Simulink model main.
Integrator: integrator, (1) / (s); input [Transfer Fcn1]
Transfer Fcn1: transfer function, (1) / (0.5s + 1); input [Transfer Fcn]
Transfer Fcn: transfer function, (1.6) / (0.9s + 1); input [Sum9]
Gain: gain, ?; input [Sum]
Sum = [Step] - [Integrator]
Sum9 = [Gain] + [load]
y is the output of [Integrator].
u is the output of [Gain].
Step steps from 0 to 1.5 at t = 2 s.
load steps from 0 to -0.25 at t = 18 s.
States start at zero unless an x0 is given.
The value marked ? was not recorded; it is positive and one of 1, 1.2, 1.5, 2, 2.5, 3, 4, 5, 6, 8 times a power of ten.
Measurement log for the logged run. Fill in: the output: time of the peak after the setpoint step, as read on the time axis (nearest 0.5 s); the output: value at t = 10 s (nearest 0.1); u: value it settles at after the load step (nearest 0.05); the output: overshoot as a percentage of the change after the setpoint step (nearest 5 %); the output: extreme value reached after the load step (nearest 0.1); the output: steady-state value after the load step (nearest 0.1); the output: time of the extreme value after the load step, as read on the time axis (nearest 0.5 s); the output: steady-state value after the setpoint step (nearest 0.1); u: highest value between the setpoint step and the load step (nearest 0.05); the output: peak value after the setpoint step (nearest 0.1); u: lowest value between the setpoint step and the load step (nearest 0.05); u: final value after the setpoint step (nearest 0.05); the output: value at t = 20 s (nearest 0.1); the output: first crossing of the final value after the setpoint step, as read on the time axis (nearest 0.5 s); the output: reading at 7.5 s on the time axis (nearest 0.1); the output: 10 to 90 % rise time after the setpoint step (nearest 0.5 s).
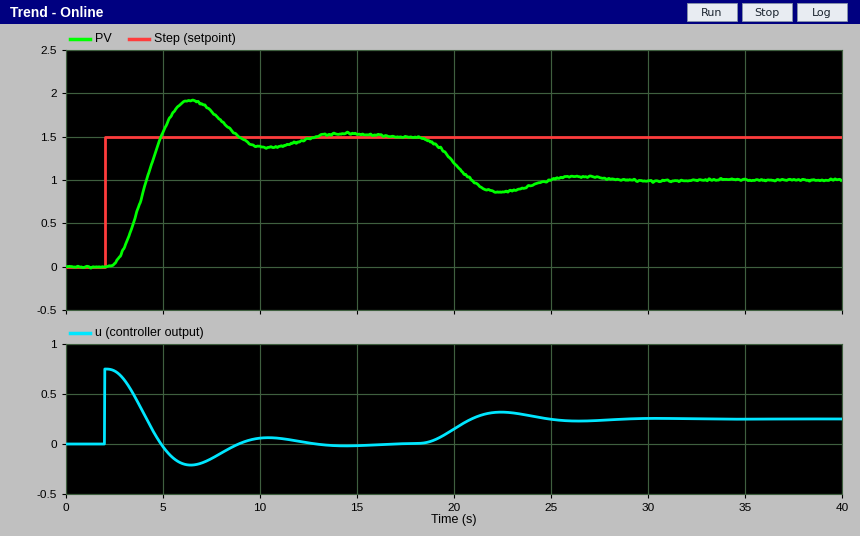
6.5 s
1.4
0.25
30 %
0.9
1.0
22.5 s
1.5
0.75
1.9
-0.20
0.00
1.2
5.0 s
1.8
2.0 s
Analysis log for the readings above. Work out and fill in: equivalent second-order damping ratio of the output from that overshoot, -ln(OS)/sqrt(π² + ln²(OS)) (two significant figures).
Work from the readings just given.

0.36
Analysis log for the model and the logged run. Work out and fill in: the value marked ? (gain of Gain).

0.5
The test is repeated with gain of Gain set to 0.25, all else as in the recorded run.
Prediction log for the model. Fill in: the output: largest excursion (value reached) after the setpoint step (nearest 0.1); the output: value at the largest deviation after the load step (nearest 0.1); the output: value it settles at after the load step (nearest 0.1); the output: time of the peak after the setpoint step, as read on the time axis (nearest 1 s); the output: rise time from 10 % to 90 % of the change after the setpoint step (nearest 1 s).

1.6
0.4
0.5
9 s
3 s
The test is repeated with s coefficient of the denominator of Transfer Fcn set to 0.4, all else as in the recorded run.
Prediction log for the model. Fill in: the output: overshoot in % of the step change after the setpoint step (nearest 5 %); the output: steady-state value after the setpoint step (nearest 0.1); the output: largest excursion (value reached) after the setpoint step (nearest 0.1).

15 %
1.5
1.7
